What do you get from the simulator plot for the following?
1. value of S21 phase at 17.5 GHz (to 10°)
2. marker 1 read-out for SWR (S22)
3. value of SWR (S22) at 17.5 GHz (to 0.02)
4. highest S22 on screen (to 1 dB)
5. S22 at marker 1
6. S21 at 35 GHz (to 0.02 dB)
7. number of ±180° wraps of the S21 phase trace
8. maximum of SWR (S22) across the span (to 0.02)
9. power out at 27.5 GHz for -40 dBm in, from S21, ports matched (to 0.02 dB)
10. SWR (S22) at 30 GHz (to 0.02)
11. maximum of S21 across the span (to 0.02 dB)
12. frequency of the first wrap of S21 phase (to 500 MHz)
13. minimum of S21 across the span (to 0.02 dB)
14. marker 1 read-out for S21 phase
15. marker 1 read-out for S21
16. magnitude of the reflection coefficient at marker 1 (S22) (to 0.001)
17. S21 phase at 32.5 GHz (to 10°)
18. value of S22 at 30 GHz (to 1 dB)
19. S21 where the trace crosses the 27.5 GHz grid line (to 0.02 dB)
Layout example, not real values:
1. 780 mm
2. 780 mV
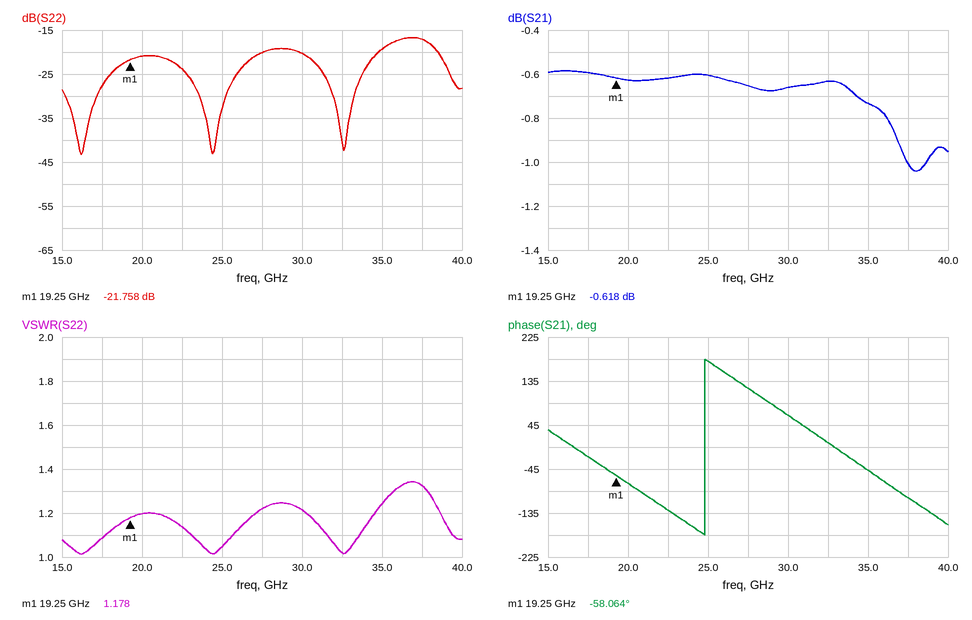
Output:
1. -20°
2. 1.178
3. 1.08
4. -17 dB
5. -21.758 dB
6. -0.74 dB
7. 1
8. 1.34
9. -40.66 dBm
10. 1.22
11. -0.58 dB
12. 25.0 GHz
13. -1.04 dB
14. -58.064°
15. -0.618 dB
16. 0.082
17. 10°
18. -20 dB
19. -0.66 dB
